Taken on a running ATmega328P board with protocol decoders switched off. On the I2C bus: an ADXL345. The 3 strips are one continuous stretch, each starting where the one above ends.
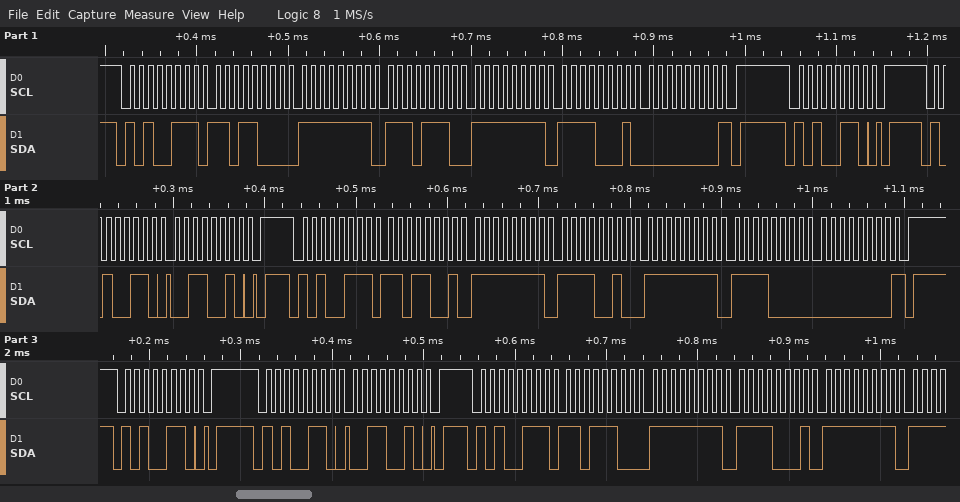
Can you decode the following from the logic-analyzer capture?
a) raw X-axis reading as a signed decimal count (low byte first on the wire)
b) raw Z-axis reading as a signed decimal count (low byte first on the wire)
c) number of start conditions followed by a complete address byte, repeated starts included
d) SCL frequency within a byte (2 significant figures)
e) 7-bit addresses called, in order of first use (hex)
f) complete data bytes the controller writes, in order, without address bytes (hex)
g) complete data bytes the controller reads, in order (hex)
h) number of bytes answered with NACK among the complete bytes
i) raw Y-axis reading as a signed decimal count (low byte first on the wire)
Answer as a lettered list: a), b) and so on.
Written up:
a) -39
b) 240
c) 7
d) 100 kHz
e) 0x53
f) 32 32
g) D8 FF EE FF F1 00 D9 FF F2 FF F0 00 DC FF F1 FF
h) 2
i) -14
